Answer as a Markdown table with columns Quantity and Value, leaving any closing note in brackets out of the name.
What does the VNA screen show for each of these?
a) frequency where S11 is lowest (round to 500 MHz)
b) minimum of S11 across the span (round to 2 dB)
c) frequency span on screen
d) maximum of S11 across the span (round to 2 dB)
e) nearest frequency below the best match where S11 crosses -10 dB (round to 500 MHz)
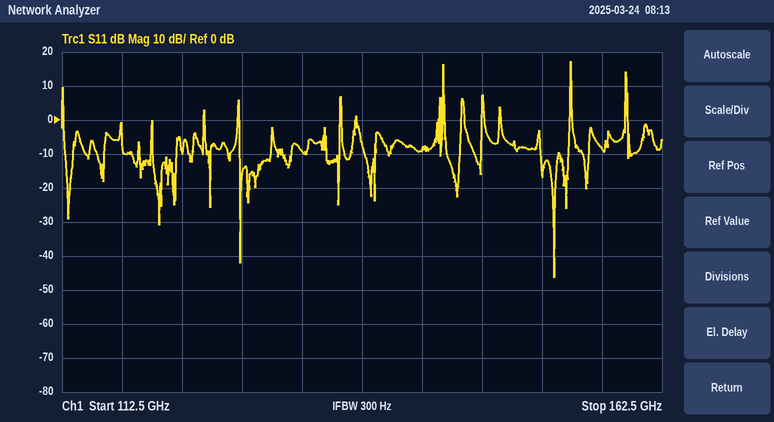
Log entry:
| Quantity | Value |
|---|---|
| frequency where S11 is lowest | 153.5 GHz |
| minimum of S11 across the span | -46 dB |
| frequency span on screen | 50 GHz |
| maximum of S11 across the span | 18 dB |
| nearest frequency below the best match where S11 crosses -10 dB | 152.5 GHz |
